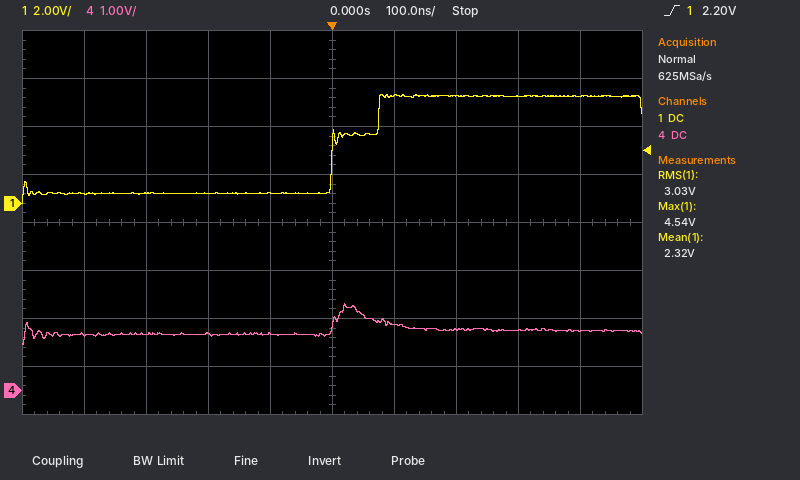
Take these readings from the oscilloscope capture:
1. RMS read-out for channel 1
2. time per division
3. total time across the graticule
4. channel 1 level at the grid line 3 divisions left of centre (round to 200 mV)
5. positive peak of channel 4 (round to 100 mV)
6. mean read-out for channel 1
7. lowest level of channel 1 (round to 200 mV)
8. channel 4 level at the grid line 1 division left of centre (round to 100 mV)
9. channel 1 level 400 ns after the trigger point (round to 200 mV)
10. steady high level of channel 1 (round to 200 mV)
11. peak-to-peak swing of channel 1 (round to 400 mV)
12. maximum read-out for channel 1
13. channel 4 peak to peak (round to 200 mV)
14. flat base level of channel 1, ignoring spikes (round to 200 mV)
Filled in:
3.03 V
100 ns
1 µs
400 mV
1.8 V
2.32 V
0.0 V
1.2 V
4.4 V
4.4 V
4.4 V
4.54 V
800 mV
400 mV
